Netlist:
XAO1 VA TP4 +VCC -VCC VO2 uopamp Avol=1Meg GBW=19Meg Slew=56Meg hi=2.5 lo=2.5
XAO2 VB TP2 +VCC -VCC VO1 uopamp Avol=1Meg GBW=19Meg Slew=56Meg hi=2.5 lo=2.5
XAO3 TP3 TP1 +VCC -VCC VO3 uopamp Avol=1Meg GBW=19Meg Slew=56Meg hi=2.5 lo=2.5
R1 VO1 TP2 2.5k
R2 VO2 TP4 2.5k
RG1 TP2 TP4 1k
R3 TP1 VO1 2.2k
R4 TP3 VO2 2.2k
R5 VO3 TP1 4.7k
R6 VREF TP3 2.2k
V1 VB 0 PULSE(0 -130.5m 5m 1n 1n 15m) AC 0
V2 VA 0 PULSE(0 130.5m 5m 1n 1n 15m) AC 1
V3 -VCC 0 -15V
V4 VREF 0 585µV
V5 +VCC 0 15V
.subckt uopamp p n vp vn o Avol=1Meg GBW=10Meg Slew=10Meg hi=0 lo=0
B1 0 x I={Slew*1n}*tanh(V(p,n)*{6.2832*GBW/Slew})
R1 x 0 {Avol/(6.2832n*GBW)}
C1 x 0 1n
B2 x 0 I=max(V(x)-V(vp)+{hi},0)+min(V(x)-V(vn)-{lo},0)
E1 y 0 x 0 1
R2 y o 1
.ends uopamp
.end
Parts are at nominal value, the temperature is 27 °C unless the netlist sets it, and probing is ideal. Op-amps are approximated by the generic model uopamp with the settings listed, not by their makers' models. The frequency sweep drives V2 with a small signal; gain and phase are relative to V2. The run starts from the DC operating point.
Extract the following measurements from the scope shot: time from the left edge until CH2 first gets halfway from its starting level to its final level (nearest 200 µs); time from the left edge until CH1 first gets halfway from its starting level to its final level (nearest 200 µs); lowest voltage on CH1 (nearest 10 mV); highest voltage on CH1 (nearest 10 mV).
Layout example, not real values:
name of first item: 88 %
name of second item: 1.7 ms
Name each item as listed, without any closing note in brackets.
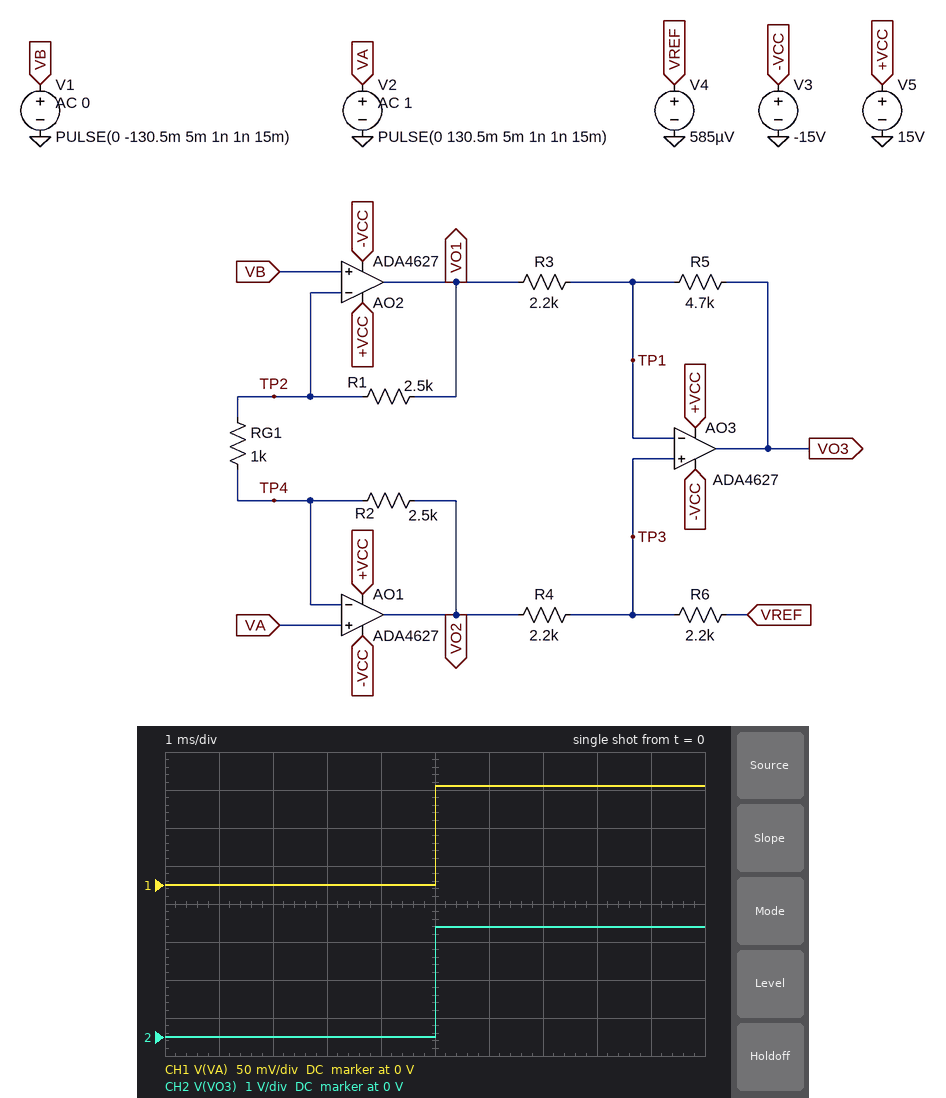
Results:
time from the left edge until CH2 first gets halfway from its starting level to its final level: 5.0 ms
time from the left edge until CH1 first gets halfway from its starting level to its final level: 5.0 ms
lowest voltage on CH1: 0 V
highest voltage on CH1: 130 mV
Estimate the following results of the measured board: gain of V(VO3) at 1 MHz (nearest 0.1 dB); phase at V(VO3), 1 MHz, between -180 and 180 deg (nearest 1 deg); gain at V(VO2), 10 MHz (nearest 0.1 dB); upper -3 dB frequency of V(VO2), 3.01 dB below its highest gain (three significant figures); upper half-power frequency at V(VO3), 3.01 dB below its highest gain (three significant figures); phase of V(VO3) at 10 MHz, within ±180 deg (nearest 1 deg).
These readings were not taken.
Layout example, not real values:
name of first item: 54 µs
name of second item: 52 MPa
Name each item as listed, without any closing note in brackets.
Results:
gain of V(VO3) at 1 MHz: 20.2 dB
phase at V(VO3), 1 MHz, between -180 and 180 deg: -27 deg
gain at V(VO2), 10 MHz: 2.0 dB
upper -3 dB frequency of V(VO2), 3.01 dB below its highest gain: 3.34 MHz
upper half-power frequency at V(VO3), 3.01 dB below its highest gain: 2.61 MHz
phase of V(VO3) at 10 MHz, within ±180 deg: -134 deg
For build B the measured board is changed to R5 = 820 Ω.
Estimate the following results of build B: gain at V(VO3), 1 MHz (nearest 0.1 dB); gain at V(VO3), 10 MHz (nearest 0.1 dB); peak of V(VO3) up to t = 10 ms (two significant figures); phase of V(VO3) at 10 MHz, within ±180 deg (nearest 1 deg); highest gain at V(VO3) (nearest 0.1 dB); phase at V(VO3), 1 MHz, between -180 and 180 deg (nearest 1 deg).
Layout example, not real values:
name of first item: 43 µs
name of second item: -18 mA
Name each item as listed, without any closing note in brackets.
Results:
gain at V(VO3), 1 MHz: 10.0 dB
gain at V(VO3), 10 MHz: -1.3 dB
peak of V(VO3) up to t = 10 ms: 830 mV
phase of V(VO3) at 10 MHz, within ±180 deg: -103 deg
highest gain at V(VO3): 10.5 dB
phase at V(VO3), 1 MHz, between -180 and 180 deg: -21 deg
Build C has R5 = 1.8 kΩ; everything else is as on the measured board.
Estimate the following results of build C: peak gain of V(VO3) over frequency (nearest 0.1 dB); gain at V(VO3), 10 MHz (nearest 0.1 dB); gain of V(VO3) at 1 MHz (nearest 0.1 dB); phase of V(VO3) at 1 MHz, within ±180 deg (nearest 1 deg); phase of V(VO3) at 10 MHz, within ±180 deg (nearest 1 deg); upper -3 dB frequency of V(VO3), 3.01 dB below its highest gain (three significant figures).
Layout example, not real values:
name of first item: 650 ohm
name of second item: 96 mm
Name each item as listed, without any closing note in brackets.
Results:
peak gain of V(VO3) over frequency: 14.4 dB
gain at V(VO3), 10 MHz: 1.2 dB
gain of V(VO3) at 1 MHz: 13.9 dB
phase of V(VO3) at 1 MHz, within ±180 deg: -23 deg
phase of V(VO3) at 10 MHz, within ±180 deg: -115 deg
upper -3 dB frequency of V(VO3), 3.01 dB below its highest gain: 2.93 MHz
